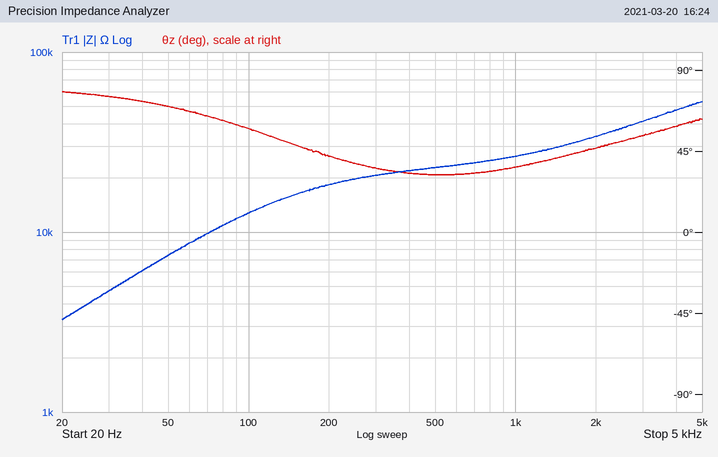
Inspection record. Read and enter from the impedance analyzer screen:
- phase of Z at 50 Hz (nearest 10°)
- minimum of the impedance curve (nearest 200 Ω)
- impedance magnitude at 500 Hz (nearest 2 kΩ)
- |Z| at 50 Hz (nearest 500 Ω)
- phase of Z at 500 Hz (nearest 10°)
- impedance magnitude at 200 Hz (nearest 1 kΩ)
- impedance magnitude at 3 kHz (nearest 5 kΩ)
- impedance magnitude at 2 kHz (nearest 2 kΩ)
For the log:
70°
3.2 kΩ
22 kΩ
7.5 kΩ
30°
18 kΩ
40 kΩ
34 kΩ
